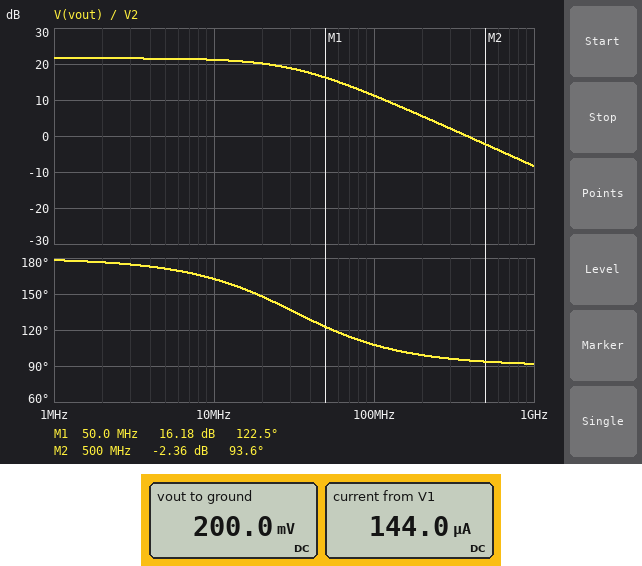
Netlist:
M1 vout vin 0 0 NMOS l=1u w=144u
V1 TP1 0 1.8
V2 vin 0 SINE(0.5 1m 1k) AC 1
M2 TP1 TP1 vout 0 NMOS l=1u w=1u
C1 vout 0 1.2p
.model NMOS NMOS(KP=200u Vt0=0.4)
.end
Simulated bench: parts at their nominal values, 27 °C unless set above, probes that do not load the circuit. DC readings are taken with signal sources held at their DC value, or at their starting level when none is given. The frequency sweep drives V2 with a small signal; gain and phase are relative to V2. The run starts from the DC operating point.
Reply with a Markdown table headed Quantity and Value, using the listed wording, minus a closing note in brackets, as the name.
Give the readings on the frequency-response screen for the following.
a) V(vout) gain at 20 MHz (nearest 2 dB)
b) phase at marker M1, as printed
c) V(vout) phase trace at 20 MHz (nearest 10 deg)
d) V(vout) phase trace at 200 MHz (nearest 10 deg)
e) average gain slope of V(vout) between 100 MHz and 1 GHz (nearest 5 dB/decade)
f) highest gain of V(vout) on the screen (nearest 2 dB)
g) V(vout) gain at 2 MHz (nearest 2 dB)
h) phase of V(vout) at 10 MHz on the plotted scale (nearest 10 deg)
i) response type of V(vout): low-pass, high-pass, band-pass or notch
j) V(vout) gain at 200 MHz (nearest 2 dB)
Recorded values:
| Quantity | Value |
|---|---|
| V(vout) gain at 20 MHz | 20 dB |
| phase at marker M1, as printed | 122.5 deg |
| V(vout) phase trace at 20 MHz | 150 deg |
| V(vout) phase trace at 200 MHz | 100 deg |
| average gain slope of V(vout) between 100 MHz and 1 GHz | -20 dB/decade |
| highest gain of V(vout) on the screen | 22 dB |
| V(vout) gain at 2 MHz | 22 dB |
| phase of V(vout) at 10 MHz on the plotted scale | 160 deg |
| response type of V(vout): low-pass, high-pass, band-pass or notch | low-pass |
| V(vout) gain at 200 MHz | 6 dB |
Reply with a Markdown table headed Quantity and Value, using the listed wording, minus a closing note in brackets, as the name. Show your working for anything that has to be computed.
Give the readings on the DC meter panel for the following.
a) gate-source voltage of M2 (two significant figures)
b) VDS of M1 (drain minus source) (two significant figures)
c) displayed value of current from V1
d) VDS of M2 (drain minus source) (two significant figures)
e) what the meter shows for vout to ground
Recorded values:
| Quantity | Value |
|---|---|
| gate-source voltage of M2 | 1.8 V - 200 mV = 1.6 V |
| VDS of M1 (drain minus source) | 200 mV = 200 mV |
| displayed value of current from V1 | 144.0 µA |
| VDS of M2 (drain minus source) | 1.8 V - 200 mV = 1.6 V |
| what the meter shows for vout to ground | 200.0 mV |
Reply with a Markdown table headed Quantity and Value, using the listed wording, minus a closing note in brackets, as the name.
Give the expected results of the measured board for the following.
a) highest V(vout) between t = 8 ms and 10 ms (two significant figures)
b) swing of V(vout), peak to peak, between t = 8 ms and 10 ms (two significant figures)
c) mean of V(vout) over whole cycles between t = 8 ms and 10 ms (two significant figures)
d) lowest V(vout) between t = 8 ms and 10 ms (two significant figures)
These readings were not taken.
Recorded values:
| Quantity | Value |
|---|---|
| highest V(vout) between t = 8 ms and 10 ms | 210 mV |
| swing of V(vout), peak to peak, between t = 8 ms and 10 ms | 24 mV |
| mean of V(vout) over whole cycles between t = 8 ms and 10 ms | 200 mV |
| lowest V(vout) between t = 8 ms and 10 ms | 190 mV |
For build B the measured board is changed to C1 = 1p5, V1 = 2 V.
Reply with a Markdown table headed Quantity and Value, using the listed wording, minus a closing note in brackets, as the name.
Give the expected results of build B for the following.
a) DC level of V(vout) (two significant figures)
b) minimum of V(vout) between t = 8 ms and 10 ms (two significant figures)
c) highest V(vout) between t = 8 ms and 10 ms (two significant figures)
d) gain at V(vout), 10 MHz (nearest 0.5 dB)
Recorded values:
| Quantity | Value |
|---|---|
| DC level of V(vout) | 400 mV |
| minimum of V(vout) between t = 8 ms and 10 ms | 390 mV |
| highest V(vout) between t = 8 ms and 10 ms | 410 mV |
| gain at V(vout), 10 MHz | 21.0 dB |
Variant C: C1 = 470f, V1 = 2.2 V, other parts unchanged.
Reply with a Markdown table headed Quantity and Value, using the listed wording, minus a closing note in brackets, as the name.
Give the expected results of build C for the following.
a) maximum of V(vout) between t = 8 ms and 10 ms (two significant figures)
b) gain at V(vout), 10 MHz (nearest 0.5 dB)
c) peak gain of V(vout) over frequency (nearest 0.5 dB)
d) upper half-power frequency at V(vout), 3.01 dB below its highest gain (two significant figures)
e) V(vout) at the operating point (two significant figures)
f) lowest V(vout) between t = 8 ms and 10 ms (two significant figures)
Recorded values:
| Quantity | Value |
|---|---|
| maximum of V(vout) between t = 8 ms and 10 ms | 610 mV |
| gain at V(vout), 10 MHz | 21.5 dB |
| peak gain of V(vout) over frequency | 21.5 dB |
| upper half-power frequency at V(vout), 3.01 dB below its highest gain | 81 MHz |
| V(vout) at the operating point | 600 mV |
| lowest V(vout) between t = 8 ms and 10 ms | 590 mV |
